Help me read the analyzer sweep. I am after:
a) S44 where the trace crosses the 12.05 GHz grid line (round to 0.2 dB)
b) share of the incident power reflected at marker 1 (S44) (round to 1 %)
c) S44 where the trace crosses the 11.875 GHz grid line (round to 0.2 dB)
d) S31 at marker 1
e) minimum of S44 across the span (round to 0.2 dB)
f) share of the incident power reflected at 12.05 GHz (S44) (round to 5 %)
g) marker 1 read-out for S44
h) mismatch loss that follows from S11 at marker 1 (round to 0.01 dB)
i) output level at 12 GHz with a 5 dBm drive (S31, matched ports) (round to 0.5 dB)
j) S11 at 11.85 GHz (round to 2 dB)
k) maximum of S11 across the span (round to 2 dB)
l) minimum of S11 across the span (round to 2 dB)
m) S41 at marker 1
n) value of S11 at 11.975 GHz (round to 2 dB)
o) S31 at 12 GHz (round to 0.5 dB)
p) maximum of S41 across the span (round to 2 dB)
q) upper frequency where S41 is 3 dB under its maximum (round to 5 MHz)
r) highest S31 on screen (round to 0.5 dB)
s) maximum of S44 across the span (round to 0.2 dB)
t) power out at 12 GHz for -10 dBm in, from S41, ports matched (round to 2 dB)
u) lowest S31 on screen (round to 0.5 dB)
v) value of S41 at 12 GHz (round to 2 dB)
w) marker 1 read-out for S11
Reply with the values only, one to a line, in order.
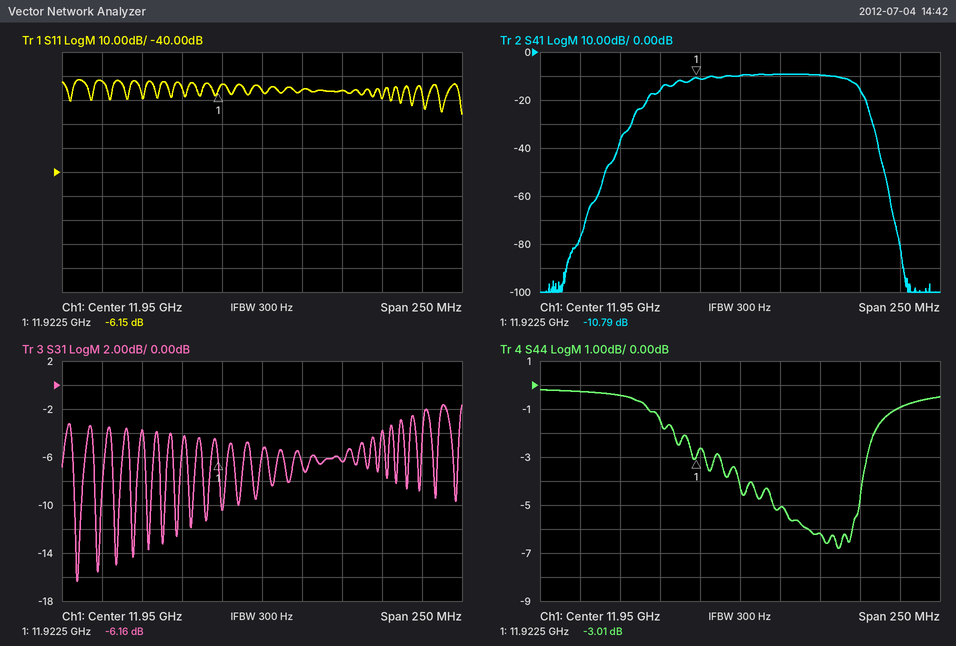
-1.0 dB
50 %
-0.4 dB
-6.16 dB
-6.8 dB
80 %
-3.01 dB
1.21 dB
-1.5 dBm
-2 dB
-2 dB
-16 dB
-10.79 dB
-6 dB
-6.5 dB
-10 dB
12.020 GHz
-1.5 dB
-0.2 dB
-20 dBm
-16.5 dB
-10 dB
-6.15 dB
